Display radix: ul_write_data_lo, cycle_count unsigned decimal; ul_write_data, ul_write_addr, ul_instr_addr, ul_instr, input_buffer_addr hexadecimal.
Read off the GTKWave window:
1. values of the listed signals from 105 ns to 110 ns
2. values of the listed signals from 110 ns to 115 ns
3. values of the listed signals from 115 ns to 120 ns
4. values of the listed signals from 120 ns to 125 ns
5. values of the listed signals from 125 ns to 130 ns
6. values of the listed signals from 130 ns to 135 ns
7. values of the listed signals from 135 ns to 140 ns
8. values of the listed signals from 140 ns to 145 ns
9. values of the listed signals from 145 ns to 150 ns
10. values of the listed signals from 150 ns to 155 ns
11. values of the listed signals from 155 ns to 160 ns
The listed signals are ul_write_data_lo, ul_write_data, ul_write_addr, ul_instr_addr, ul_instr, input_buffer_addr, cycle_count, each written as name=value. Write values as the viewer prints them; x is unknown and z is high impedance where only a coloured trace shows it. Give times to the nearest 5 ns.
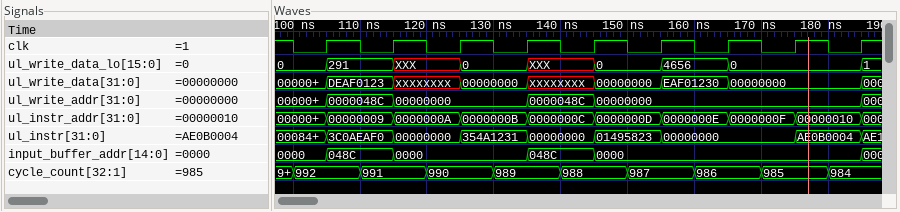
ul_write_data_lo=291, ul_write_data=DEAF0123, ul_write_addr=0000048C, ul_instr_addr=00000009, ul_instr=3C0AEAF0, input_buffer_addr=048C, cycle_count=992
ul_write_data_lo=291, ul_write_data=DEAF0123, ul_write_addr=0000048C, ul_instr_addr=00000009, ul_instr=3C0AEAF0, input_buffer_addr=048C, cycle_count=991
ul_write_data_lo=XXX, ul_write_data=xxxxxxxx, ul_write_addr=00000000, ul_instr_addr=0000000A, ul_instr=00000000, input_buffer_addr=0000, cycle_count=991
ul_write_data_lo=XXX, ul_write_data=xxxxxxxx, ul_write_addr=00000000, ul_instr_addr=0000000A, ul_instr=00000000, input_buffer_addr=0000, cycle_count=990
ul_write_data_lo=0, ul_write_data=00000000, ul_write_addr=00000000, ul_instr_addr=0000000B, ul_instr=354A1231, input_buffer_addr=0000, cycle_count=990
ul_write_data_lo=0, ul_write_data=00000000, ul_write_addr=00000000, ul_instr_addr=0000000B, ul_instr=354A1231, input_buffer_addr=0000, cycle_count=989
ul_write_data_lo=XXX, ul_write_data=xxxxxxxx, ul_write_addr=0000048C, ul_instr_addr=0000000C, ul_instr=00000000, input_buffer_addr=048C, cycle_count=989
ul_write_data_lo=XXX, ul_write_data=xxxxxxxx, ul_write_addr=0000048C, ul_instr_addr=0000000C, ul_instr=00000000, input_buffer_addr=048C, cycle_count=988
ul_write_data_lo=0, ul_write_data=00000000, ul_write_addr=00000000, ul_instr_addr=0000000D, ul_instr=01495823, input_buffer_addr=0000, cycle_count=988
ul_write_data_lo=0, ul_write_data=00000000, ul_write_addr=00000000, ul_instr_addr=0000000D, ul_instr=01495823, input_buffer_addr=0000, cycle_count=987
ul_write_data_lo=4656, ul_write_data=EAF01230, ul_write_addr=00000000, ul_instr_addr=0000000E, ul_instr=00000000, input_buffer_addr=0000, cycle_count=987
